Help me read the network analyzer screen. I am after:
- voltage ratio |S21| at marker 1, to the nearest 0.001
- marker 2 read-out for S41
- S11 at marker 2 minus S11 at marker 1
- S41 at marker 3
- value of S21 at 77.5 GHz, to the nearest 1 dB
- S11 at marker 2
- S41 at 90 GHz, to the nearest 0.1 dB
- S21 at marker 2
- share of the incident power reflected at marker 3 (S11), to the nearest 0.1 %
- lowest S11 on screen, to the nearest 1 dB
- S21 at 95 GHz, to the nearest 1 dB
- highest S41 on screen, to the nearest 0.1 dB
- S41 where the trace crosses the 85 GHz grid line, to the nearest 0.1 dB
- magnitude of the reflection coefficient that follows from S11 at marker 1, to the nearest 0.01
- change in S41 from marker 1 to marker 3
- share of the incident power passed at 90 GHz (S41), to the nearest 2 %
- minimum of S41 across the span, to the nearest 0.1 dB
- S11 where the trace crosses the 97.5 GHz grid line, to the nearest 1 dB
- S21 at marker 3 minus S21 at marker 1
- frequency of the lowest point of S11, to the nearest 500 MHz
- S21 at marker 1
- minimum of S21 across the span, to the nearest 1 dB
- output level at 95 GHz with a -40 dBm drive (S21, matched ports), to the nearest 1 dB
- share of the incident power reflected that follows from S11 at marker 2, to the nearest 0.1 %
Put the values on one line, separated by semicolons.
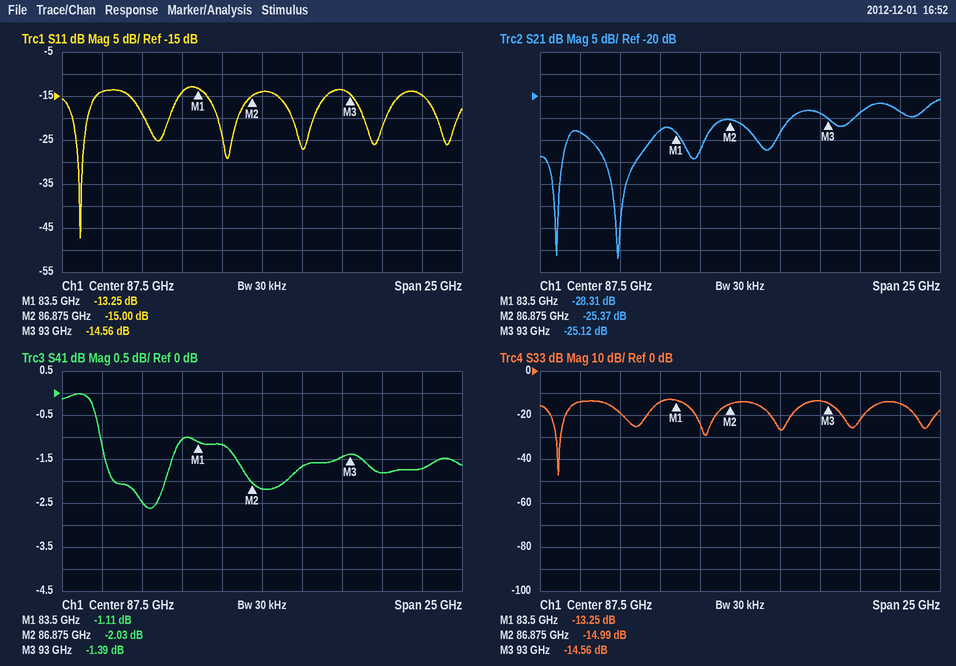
0.038; -2.03 dB; -1.75 dB; -1.39 dB; -28 dB; -15.00 dB; -1.7 dB; -25.37 dB; 3.5 %; -47 dB; -24 dB; 0.0 dB; -1.2 dB; 0.22; -0.28 dB; 68 %; -2.6 dB; -15 dB; 3.19 dB; 76.0 GHz; -28.31 dB; -57 dB; -64 dBm; 3.2 %
